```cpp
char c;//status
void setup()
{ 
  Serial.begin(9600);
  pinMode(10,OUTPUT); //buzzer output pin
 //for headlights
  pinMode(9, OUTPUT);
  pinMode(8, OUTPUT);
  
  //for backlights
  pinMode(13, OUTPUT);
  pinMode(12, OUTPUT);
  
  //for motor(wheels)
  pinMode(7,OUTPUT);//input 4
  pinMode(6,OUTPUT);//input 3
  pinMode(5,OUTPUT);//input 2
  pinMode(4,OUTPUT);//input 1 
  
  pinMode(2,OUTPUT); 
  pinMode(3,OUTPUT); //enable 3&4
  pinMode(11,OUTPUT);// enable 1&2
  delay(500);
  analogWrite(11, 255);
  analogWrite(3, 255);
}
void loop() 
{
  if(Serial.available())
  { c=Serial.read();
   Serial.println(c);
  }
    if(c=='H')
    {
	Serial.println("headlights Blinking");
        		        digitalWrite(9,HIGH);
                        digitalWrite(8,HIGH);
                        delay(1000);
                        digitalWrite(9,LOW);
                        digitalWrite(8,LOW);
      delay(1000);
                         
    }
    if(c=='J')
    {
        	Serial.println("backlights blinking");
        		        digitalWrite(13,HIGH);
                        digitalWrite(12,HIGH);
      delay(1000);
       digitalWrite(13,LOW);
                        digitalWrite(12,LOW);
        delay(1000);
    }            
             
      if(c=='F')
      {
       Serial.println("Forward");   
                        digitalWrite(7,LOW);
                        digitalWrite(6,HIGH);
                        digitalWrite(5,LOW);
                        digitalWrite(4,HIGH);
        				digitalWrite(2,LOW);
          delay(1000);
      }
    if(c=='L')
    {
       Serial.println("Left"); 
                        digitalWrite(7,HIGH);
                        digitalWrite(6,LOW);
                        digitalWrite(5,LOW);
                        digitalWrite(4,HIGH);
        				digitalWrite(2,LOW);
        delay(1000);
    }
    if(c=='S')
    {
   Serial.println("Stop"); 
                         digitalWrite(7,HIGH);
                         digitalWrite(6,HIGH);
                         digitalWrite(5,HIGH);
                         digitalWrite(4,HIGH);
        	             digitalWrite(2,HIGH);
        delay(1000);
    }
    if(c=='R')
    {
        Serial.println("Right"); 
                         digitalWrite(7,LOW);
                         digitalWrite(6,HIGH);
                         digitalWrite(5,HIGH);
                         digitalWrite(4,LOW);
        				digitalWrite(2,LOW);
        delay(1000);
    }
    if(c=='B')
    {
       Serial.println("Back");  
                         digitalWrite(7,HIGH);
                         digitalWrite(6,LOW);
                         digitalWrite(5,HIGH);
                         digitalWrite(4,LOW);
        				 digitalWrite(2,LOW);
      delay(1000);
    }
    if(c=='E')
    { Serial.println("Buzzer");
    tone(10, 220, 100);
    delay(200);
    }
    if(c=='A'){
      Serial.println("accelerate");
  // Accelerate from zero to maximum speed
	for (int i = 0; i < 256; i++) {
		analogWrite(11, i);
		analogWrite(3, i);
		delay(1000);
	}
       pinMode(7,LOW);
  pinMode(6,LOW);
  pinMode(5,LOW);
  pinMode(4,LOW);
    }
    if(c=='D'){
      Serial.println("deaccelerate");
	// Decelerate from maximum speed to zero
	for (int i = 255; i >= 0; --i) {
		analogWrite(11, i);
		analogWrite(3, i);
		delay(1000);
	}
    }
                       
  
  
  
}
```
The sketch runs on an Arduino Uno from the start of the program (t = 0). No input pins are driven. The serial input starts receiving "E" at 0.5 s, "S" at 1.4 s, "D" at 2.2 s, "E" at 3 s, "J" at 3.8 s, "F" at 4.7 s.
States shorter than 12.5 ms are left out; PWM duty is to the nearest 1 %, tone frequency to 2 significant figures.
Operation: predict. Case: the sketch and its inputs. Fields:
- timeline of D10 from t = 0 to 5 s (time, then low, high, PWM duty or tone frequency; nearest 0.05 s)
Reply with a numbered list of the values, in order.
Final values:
1. 0 s low; 0.5 s tone 220 Hz; 0.6 s low; 0.7 s tone 220 Hz; 0.8 s low; 0.9 s tone 220 Hz; 1 s low; 1.1 s tone 220 Hz; 1.2 s low; 1.3 s tone 220 Hz; 1.4 s low
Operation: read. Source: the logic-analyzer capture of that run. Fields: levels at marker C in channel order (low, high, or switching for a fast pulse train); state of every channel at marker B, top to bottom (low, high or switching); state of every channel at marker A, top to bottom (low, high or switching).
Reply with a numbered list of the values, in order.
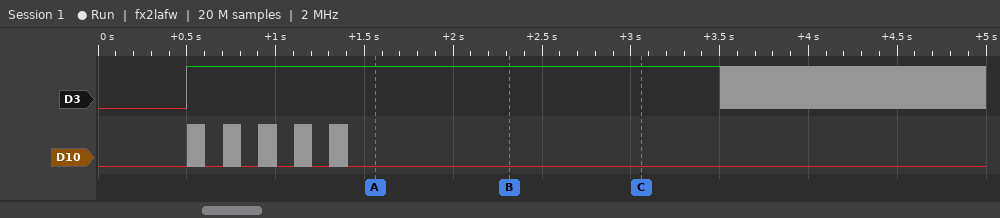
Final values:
1. D3 high, D10 low
2. D3 high, D10 low
3. D3 high, D10 low
